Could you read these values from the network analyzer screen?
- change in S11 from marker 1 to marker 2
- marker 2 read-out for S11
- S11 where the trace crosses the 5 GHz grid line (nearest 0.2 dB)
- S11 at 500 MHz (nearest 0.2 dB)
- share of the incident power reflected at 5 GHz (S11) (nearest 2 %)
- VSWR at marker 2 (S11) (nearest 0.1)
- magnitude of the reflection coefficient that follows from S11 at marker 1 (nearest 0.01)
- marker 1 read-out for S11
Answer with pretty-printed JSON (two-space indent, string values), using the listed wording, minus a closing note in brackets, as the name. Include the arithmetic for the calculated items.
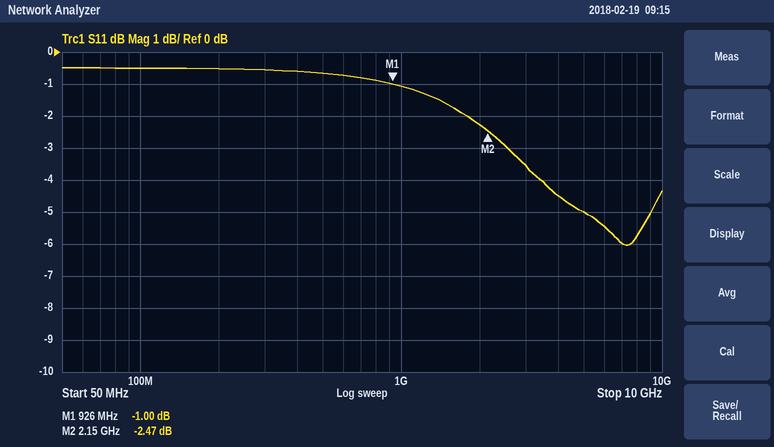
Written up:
{
  "change in S11 from marker 1 to marker 2": "-2.47 − (-1) = -1.47 dB",
  "marker 2 read-out for S11": "-2.47 dB",
  "S11 where the trace crosses the 5 GHz grid line": "-5.0 dB",
  "S11 at 500 MHz": "-0.6 dB",
  "share of the incident power reflected at 5 GHz (S11)": "10^(-5/10) ≈ 32 %",
  "VSWR at marker 2 (S11)": "(1 + 0.7525)/(1 − 0.7525) ≈ 7.1",
  "magnitude of the reflection coefficient that follows from S11 at marker 1": "10^(-1/20) ≈ 0.89",
  "marker 1 read-out for S11": "-1.00 dB"
}
